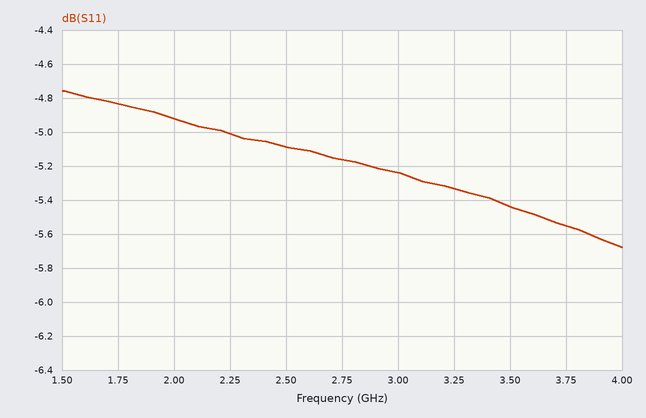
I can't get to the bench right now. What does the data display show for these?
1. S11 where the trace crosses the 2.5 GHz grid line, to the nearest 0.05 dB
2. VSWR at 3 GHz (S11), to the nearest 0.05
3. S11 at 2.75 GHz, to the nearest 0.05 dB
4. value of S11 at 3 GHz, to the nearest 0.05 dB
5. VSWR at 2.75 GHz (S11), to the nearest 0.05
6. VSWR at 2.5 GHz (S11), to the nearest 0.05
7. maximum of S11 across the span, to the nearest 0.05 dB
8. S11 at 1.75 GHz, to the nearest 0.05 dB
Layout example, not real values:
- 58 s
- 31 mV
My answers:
- -5.10 dB
- 3.40
- -5.15 dB
- -5.25 dB
- 3.45
- 3.50
- -4.75 dB
- -4.85 dB
